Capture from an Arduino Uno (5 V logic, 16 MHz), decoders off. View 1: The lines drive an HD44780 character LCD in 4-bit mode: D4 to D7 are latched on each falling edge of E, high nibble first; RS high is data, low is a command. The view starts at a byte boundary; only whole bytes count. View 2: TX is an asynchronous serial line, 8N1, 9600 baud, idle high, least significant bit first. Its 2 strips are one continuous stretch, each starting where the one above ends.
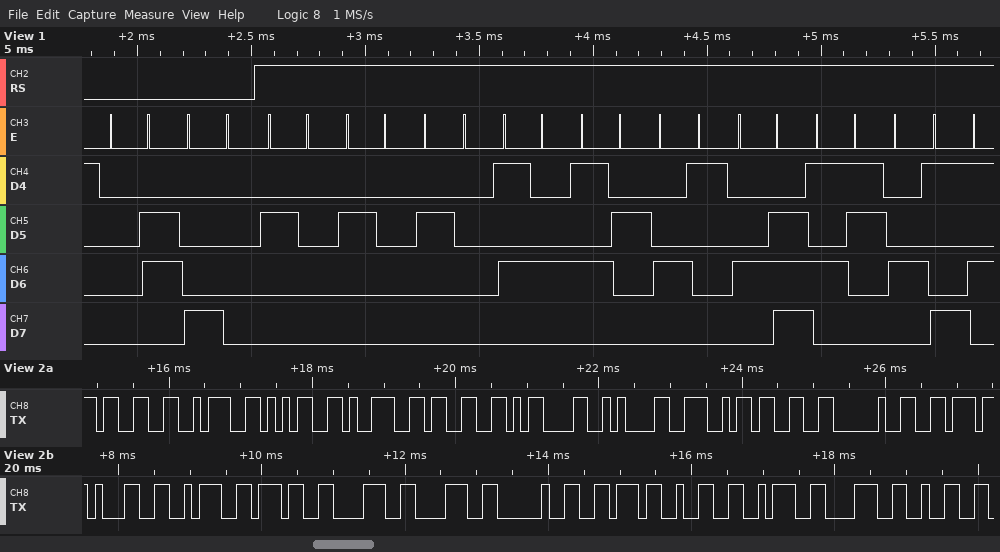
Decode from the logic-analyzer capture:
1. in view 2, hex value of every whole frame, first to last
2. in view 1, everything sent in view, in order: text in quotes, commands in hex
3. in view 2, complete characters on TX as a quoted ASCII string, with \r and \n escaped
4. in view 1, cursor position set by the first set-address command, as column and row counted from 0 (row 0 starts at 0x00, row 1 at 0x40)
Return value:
33 3A 35 39 33 0D 0A 4E 33 20 76 31 3A 37 38 38 20 76 32 3A 38 32
0x06 0x80 "   TRANSI"
"3:593\r\nN3 v1:788 v2:82"
column 0, row 0
